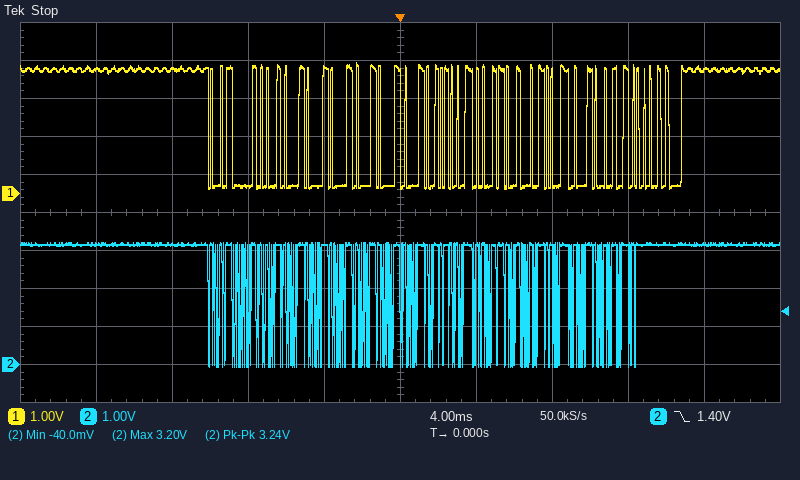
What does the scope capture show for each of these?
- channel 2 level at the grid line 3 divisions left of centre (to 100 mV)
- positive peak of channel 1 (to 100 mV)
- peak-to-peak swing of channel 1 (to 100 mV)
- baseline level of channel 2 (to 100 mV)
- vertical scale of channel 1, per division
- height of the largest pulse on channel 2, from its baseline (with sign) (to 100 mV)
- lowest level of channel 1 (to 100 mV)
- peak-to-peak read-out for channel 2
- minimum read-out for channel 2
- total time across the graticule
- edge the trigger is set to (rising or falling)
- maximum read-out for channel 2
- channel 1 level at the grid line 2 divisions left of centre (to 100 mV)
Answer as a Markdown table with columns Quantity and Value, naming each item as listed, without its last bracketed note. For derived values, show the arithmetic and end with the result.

| Quantity | Value |
|---|---|
| channel 2 level at the grid line 3 divisions left of centre | 3.2 V |
| positive peak of channel 1 | 3.4 V |
| peak-to-peak swing of channel 1 | 3.4 V − (100 mV) = 3.3 V |
| baseline level of channel 2 | 3.2 V |
| vertical scale of channel 1, per division | 1 V |
| height of the largest pulse on channel 2, from its baseline (with sign) | -3.2 V |
| lowest level of channel 1 | 100 mV |
| peak-to-peak read-out for channel 2 | 3.24 V |
| minimum read-out for channel 2 | -40.0 mV |
| total time across the graticule | 40 ms |
| edge the trigger is set to | falling |
| maximum read-out for channel 2 | 3.20 V |
| channel 1 level at the grid line 2 divisions left of centre | 200 mV |
